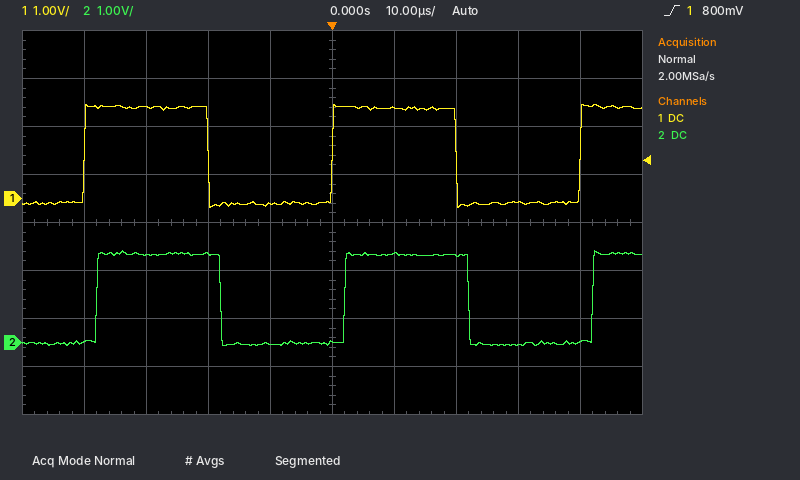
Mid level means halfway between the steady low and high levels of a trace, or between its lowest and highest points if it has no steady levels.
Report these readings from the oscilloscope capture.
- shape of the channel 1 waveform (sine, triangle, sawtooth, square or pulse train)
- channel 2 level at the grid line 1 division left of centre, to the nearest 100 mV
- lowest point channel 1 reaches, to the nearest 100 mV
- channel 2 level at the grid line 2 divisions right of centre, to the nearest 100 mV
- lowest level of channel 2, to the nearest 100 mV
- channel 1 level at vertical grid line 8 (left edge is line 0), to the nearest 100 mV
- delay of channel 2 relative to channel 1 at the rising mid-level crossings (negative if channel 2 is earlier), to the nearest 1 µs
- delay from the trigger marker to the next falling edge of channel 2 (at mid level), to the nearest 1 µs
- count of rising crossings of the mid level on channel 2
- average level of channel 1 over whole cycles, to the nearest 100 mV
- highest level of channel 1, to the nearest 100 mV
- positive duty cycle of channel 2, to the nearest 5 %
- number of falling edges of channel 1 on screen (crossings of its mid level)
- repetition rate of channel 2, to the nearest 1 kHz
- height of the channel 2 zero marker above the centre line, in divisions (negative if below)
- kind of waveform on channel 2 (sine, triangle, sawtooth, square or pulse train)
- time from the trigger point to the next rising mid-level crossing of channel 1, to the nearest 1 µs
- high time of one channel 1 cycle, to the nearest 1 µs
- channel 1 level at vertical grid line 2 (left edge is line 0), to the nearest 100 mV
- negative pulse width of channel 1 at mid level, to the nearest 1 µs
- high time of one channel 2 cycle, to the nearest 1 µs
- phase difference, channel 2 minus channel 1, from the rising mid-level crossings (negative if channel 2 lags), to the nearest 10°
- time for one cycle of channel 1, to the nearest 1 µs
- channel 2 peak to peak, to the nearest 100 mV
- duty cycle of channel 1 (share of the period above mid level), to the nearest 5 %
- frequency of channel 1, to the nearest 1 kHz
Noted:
square
0.0 V
-200 mV
1.8 V
-100 mV
-100 mV
+2 µs
22 µs
3
900 mV
2.0 V
50 %
2
25 kHz
-2.5 div
square
40 µs
20 µs
1.9 V
20 µs
20 µs
-20°
40 µs
2.0 V
50 %
25 kHz
